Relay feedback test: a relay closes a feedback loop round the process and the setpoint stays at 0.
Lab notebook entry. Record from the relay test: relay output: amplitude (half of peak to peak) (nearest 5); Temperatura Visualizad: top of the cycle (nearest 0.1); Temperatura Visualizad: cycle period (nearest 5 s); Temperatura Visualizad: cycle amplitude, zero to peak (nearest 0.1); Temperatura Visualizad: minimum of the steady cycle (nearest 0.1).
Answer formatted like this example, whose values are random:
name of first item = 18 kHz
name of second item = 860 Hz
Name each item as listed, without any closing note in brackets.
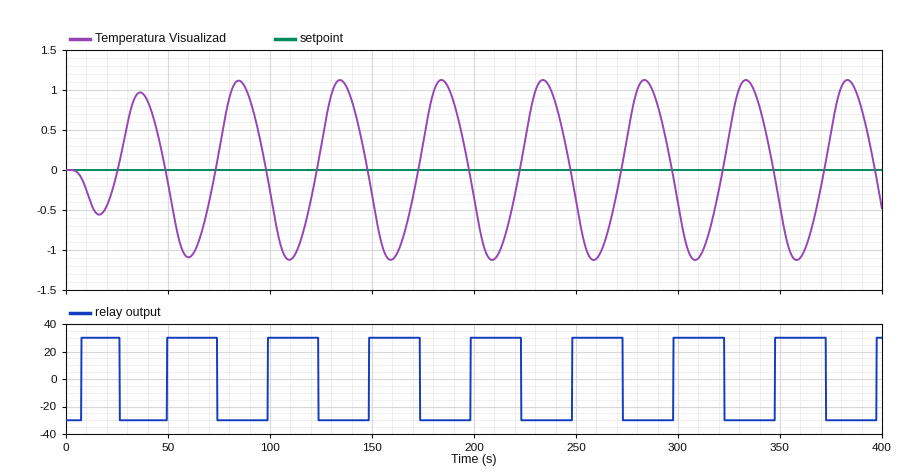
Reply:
relay output: amplitude (half of peak to peak) = 30
Temperatura Visualizad: top of the cycle = 1.1
Temperatura Visualizad: cycle period = 50 s
Temperatura Visualizad: cycle amplitude, zero to peak = 1.1
Temperatura Visualizad: minimum of the steady cycle = -1.1
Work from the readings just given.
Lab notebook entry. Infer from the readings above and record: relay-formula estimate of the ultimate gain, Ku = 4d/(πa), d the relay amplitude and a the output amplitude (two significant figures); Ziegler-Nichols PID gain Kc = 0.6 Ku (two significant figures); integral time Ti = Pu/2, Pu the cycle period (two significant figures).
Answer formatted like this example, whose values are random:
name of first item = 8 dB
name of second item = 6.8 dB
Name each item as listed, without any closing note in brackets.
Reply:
relay-formula estimate of the ultimate gain, Ku = 4d/(πa), d the relay amplitude and a the output amplitude = 35
Ziegler-Nichols PID gain Kc = 0.6 Ku = 21
integral time Ti = Pu/2, Pu the cycle period = 25 s
